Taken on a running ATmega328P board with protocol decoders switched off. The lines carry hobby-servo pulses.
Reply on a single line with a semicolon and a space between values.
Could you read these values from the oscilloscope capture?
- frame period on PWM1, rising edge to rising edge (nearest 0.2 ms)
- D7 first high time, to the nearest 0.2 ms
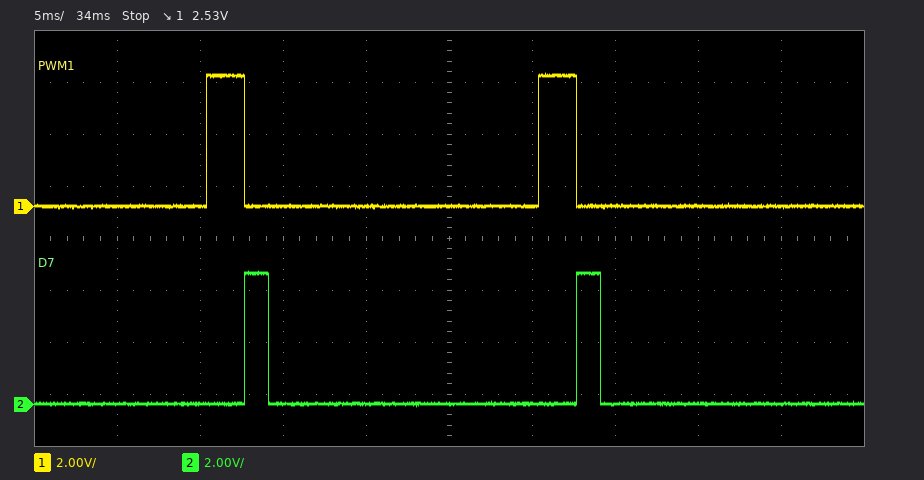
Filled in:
20.0 ms; 1.4 ms
